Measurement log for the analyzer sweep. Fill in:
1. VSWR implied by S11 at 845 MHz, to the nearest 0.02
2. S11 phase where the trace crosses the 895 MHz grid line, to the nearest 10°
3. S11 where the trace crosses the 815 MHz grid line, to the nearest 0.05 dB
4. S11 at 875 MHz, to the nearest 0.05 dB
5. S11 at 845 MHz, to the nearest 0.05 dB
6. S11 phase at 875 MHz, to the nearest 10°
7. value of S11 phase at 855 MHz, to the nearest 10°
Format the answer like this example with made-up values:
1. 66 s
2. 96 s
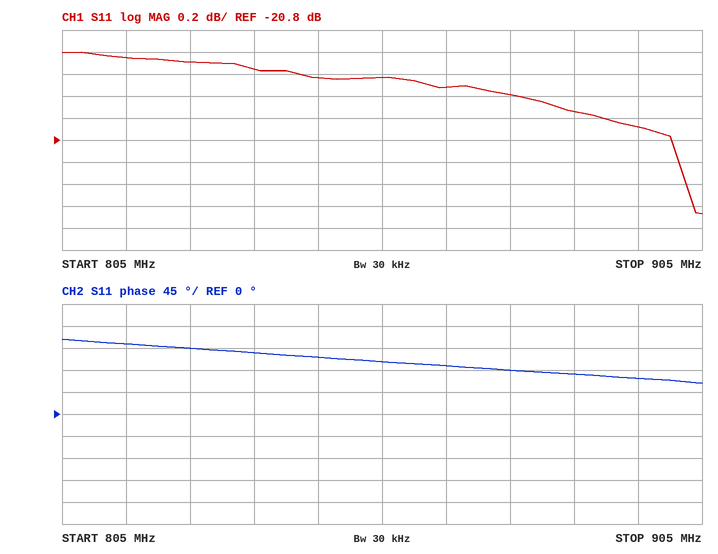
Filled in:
1. 1.22
2. 70°
3. -20.05 dB
4. -20.40 dB
5. -20.25 dB
6. 90°
7. 110°
